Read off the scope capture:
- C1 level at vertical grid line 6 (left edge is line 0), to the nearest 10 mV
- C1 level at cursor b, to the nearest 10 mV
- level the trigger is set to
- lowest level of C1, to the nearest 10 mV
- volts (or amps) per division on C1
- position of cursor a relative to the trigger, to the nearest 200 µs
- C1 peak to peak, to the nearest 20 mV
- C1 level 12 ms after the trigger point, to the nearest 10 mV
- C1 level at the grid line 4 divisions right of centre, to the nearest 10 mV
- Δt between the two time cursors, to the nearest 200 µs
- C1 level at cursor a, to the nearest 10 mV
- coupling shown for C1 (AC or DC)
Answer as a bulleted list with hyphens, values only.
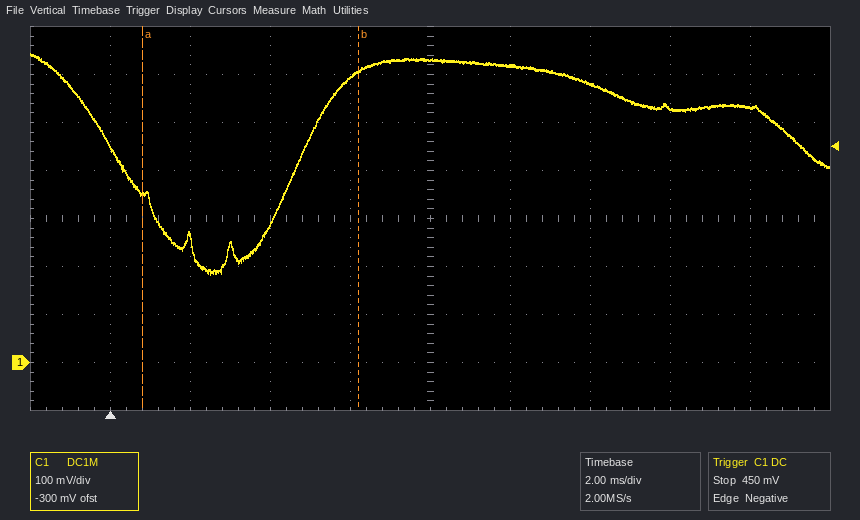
- 620 mV
- 610 mV
- 450 mV
- 180 mV
- 100 mV
- +800 µs
- 460 mV
- 580 mV
- 530 mV
- 5.4 ms
- 350 mV
- DC
